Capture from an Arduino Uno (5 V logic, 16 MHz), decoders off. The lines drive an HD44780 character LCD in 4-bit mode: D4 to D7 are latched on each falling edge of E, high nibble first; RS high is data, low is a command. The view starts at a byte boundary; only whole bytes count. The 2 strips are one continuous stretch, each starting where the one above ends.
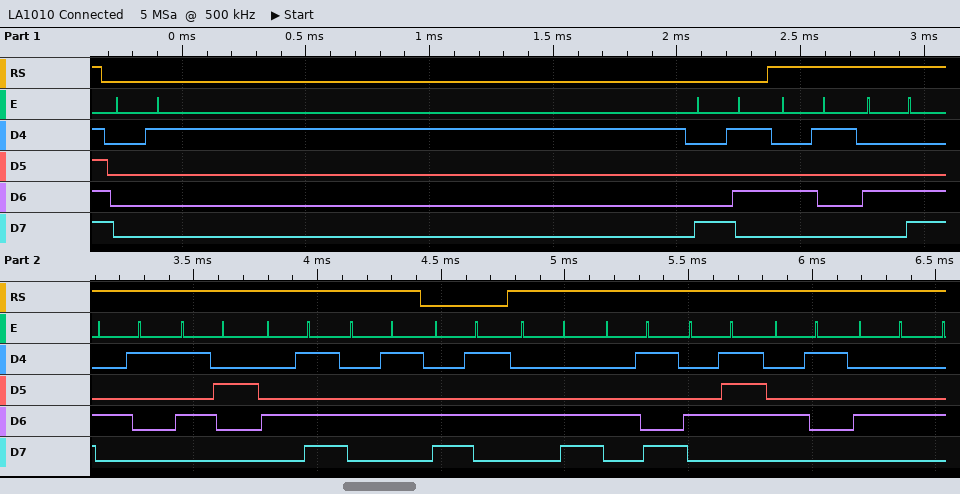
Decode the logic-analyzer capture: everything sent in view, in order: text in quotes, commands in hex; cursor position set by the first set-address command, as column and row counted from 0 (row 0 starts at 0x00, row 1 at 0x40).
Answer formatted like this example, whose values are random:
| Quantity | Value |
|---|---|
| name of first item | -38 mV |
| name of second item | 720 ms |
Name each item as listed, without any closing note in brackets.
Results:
| Quantity | Value |
|---|---|
| everything sent in view, in order: text in quotes, commands in hex | 0x01 0x85 "ALARME" 0xC5 "LIGAD" |
| cursor position set by the first set-address command, as column and row counted from 0 | column 5, row 0 |
